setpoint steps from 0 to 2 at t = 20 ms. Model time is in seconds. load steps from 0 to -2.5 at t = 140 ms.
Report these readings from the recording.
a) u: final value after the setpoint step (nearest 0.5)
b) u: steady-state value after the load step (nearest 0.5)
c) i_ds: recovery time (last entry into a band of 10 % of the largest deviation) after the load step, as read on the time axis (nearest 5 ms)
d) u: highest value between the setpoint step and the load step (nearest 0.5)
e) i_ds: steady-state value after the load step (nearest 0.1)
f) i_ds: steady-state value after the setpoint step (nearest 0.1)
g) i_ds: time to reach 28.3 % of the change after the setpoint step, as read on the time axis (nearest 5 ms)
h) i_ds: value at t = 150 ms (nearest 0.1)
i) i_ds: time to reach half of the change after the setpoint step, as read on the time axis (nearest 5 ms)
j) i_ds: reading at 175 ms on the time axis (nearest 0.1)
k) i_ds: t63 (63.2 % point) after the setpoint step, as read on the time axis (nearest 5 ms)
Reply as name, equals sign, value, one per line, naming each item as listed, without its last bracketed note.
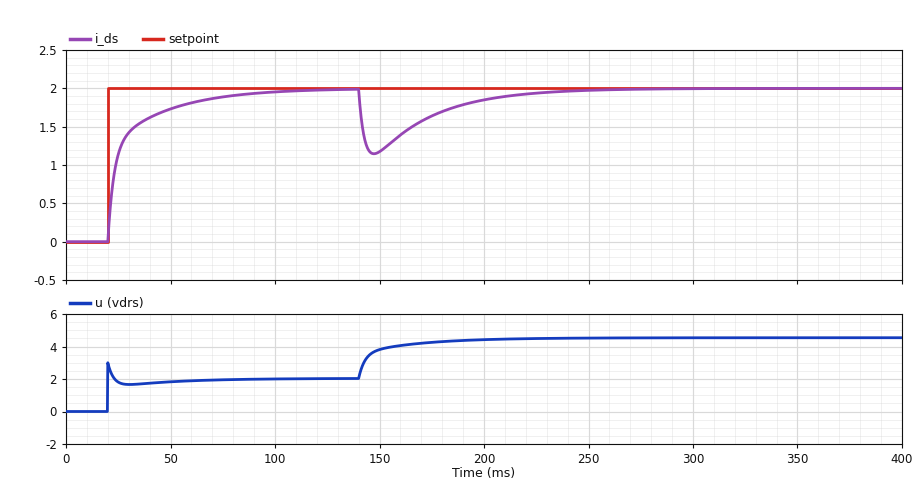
u: final value after the setpoint step = 2.0
u: steady-state value after the load step = 4.5
i_ds: recovery time (last entry into a band of 10 % of the largest deviation) after the load step, as read on the time axis = 215 ms
u: highest value between the setpoint step and the load step = 3.0
i_ds: steady-state value after the load step = 2.0
i_ds: steady-state value after the setpoint step = 2.0
i_ds: time to reach 28.3 % of the change after the setpoint step, as read on the time axis = 20 ms
i_ds: value at t = 150 ms = 1.2
i_ds: time to reach half of the change after the setpoint step, as read on the time axis = 25 ms
i_ds: reading at 175 ms on the time axis = 1.6
i_ds: t63 (63.2 % point) after the setpoint step, as read on the time axis = 25 ms
